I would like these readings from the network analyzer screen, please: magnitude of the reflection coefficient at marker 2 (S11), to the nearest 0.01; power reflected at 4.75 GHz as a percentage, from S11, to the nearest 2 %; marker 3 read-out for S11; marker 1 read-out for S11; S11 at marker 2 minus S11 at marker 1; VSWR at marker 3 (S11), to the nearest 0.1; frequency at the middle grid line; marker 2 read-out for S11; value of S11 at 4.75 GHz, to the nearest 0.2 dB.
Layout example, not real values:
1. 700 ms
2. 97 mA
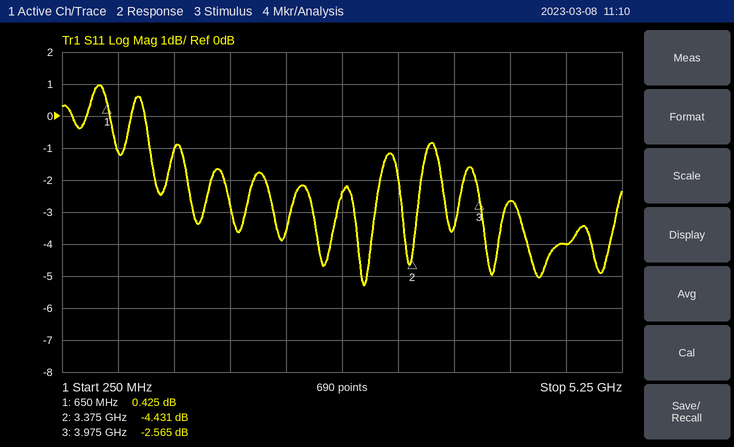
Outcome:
1. 0.60
2. 40 %
3. -2.565 dB
4. 0.425 dB
5. -4.856 dB
6. 6.8
7. 2.75 GHz
8. -4.431 dB
9. -4.0 dB
